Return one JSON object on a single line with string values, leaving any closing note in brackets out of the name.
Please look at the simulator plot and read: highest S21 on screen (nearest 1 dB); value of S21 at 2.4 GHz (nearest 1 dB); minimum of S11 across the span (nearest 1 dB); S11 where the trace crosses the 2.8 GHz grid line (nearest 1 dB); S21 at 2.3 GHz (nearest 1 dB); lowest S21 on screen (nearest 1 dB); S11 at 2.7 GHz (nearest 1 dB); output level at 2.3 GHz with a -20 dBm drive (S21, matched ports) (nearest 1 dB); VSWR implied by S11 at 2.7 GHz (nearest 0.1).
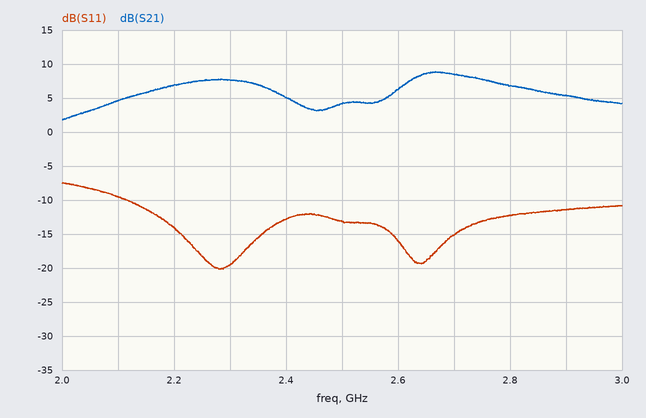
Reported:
{"highest S21 on screen": "9 dB", "value of S21 at 2.4 GHz": "5 dB", "minimum of S11 across the span": "-20 dB", "S11 where the trace crosses the 2.8 GHz grid line": "-12 dB", "S21 at 2.3 GHz": "8 dB", "lowest S21 on screen": "2 dB", "S11 at 2.7 GHz": "-15 dB", "output level at 2.3 GHz with a -20 dBm drive (S21, matched ports)": "-12 dBm", "VSWR implied by S11 at 2.7 GHz": "1.4"}
